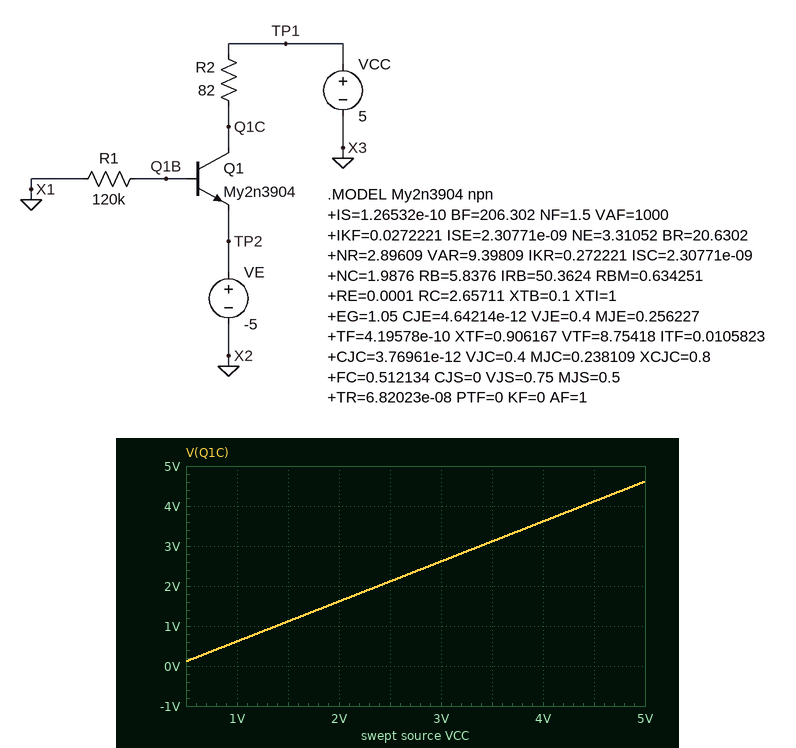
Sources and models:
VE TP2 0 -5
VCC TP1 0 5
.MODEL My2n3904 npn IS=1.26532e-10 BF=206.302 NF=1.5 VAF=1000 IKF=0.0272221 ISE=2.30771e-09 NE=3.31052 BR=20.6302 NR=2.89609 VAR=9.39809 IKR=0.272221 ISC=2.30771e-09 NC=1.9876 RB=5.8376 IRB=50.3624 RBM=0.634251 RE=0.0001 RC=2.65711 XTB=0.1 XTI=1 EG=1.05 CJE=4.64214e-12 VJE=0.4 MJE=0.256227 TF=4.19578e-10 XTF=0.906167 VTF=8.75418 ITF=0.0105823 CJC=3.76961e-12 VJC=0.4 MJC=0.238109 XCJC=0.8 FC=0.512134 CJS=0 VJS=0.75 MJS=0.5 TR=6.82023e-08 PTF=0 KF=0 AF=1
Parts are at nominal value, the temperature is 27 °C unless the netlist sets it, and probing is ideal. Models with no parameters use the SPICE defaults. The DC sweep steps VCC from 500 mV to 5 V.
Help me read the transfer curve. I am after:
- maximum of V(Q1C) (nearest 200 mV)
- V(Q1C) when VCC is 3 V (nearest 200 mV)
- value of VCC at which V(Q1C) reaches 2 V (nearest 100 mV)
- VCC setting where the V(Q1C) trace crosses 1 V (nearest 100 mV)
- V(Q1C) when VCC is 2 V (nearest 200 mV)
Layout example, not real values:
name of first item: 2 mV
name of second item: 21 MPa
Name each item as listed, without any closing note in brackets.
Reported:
maximum of V(Q1C): 4.6 V
V(Q1C) when VCC is 3 V: 2.6 V
value of VCC at which V(Q1C) reaches 2 V: 2.4 V
VCC setting where the V(Q1C) trace crosses 1 V: 1.4 V
V(Q1C) when VCC is 2 V: 1.6 V
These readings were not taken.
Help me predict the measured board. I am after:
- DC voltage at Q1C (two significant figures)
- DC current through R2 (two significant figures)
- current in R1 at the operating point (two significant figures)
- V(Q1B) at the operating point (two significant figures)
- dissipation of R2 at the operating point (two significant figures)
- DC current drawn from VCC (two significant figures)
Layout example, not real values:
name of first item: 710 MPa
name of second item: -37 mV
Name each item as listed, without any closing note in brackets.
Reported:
DC voltage at Q1C: 4.6 V
DC current through R2: 4.7 mA
current in R1 at the operating point: 36 µA
V(Q1B) at the operating point: -4.3 V
dissipation of R2 at the operating point: 1.8 mW
DC current drawn from VCC: 4.7 mA
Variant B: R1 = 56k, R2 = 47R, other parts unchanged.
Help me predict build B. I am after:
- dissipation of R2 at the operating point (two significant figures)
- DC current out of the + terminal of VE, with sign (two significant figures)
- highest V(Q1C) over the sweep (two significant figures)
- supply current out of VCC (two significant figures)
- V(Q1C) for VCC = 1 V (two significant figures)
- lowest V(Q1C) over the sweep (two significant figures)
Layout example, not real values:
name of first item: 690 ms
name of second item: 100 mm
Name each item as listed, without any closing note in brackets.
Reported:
dissipation of R2 at the operating point: 4.1 mW
DC current out of the + terminal of VE, with sign: -9.4 mA
highest V(Q1C) over the sweep: 4.6 V
supply current out of VCC: 9.3 mA
V(Q1C) for VCC = 1 V: 560 mV
lowest V(Q1C) over the sweep: 63 mV
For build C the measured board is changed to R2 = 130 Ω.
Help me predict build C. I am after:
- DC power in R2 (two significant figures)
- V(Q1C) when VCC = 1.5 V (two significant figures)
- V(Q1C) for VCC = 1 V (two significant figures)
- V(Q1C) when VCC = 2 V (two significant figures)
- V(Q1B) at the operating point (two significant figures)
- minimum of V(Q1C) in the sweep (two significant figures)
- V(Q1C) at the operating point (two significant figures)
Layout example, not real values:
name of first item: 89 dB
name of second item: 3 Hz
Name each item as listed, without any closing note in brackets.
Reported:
DC power in R2: 2.9 mW
V(Q1C) when VCC = 1.5 V: 890 mV
V(Q1C) for VCC = 1 V: 390 mV
V(Q1C) when VCC = 2 V: 1.4 V
V(Q1B) at the operating point: -4.3 V
minimum of V(Q1C) in the sweep: -110 mV
V(Q1C) at the operating point: 4.4 V
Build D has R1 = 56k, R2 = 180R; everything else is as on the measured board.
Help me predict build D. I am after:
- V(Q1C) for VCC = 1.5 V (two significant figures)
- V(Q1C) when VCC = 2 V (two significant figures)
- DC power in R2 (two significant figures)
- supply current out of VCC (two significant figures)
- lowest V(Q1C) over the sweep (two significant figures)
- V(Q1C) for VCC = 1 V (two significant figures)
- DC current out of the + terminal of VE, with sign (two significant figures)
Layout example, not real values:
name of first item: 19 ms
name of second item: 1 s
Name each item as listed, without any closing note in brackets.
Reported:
V(Q1C) for VCC = 1.5 V: -170 mV
V(Q1C) when VCC = 2 V: 330 mV
DC power in R2: 16 mW
supply current out of VCC: 9.3 mA
lowest V(Q1C) over the sweep: -1.2 V
V(Q1C) for VCC = 1 V: -670 mV
DC current out of the + terminal of VE, with sign: -9.4 mA
